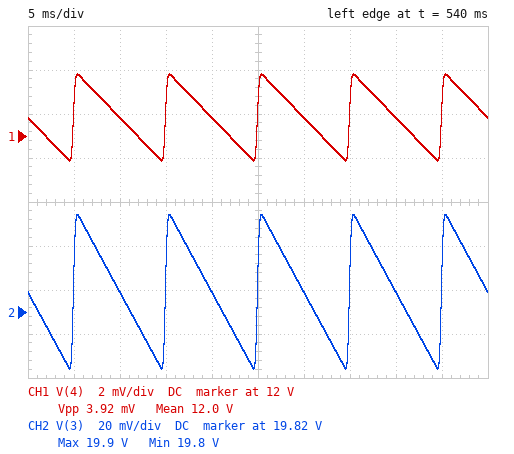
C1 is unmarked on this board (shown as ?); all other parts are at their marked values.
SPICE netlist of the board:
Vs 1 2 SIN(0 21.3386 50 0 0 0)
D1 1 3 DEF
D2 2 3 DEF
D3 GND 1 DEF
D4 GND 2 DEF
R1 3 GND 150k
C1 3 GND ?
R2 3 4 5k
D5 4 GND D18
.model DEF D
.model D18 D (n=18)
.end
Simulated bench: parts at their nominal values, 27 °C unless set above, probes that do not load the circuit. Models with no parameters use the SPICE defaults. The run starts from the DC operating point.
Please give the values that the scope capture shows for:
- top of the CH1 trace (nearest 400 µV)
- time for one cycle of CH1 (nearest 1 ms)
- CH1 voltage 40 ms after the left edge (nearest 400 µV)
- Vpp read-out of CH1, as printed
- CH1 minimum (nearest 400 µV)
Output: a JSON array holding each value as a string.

["12.0028 V", "10 ms", "12.0008 V", "3.92 mV", "11.9988 V"]
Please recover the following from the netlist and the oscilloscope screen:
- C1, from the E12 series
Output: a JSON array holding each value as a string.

["220 µF"]
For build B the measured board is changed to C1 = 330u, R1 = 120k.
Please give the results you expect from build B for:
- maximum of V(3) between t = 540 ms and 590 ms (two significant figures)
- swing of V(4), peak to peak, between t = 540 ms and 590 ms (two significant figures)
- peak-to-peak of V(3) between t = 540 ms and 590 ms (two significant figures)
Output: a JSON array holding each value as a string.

["20 V", "2.7 mV", "48 mV"]
